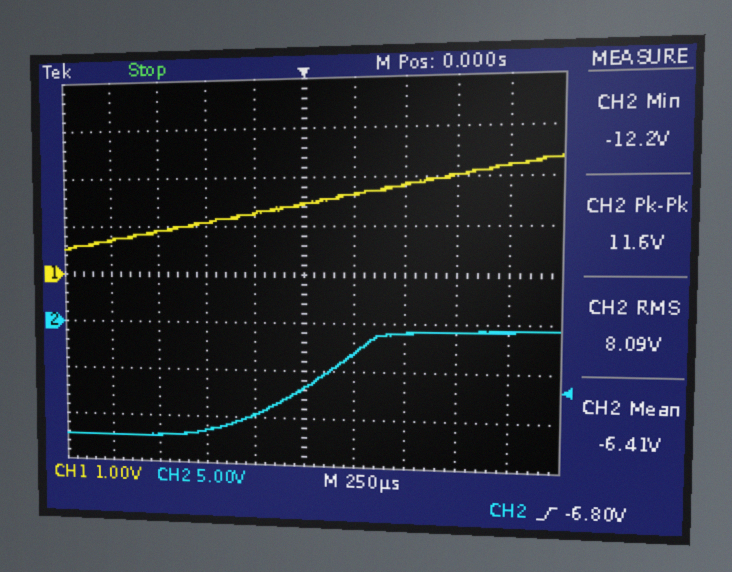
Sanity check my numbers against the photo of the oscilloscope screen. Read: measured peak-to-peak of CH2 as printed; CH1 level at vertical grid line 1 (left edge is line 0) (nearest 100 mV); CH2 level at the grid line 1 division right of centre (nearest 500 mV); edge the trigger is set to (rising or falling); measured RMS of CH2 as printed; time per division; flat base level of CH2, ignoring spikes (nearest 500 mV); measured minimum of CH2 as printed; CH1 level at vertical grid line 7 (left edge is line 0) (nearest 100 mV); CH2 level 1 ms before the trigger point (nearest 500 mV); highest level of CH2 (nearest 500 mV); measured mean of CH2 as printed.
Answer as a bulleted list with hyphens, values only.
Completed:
- 11.6 V
- 700 mV
- -3.0 V
- rising
- 8.09 V
- 250 µs
- -12.0 V
- -12.2 V
- 1.8 V
- -12.0 V
- -500 mV
- -6.41 V
